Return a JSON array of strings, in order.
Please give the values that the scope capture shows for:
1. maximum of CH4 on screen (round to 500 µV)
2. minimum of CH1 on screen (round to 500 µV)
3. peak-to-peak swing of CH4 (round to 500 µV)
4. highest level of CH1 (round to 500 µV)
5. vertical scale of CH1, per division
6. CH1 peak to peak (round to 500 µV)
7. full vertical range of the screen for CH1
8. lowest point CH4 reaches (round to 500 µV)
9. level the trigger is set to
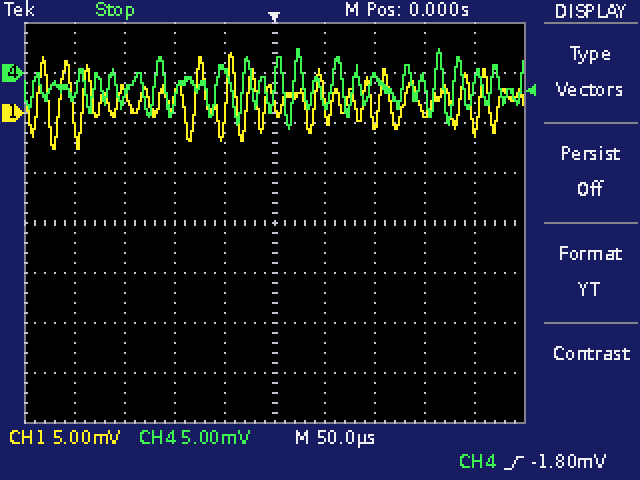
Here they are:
["2.5 mV", "-3.5 mV", "8.0 mV", "6.0 mV", "5 mV", "9.5 mV", "40 mV", "-5.5 mV", "-1.80 mV"]
